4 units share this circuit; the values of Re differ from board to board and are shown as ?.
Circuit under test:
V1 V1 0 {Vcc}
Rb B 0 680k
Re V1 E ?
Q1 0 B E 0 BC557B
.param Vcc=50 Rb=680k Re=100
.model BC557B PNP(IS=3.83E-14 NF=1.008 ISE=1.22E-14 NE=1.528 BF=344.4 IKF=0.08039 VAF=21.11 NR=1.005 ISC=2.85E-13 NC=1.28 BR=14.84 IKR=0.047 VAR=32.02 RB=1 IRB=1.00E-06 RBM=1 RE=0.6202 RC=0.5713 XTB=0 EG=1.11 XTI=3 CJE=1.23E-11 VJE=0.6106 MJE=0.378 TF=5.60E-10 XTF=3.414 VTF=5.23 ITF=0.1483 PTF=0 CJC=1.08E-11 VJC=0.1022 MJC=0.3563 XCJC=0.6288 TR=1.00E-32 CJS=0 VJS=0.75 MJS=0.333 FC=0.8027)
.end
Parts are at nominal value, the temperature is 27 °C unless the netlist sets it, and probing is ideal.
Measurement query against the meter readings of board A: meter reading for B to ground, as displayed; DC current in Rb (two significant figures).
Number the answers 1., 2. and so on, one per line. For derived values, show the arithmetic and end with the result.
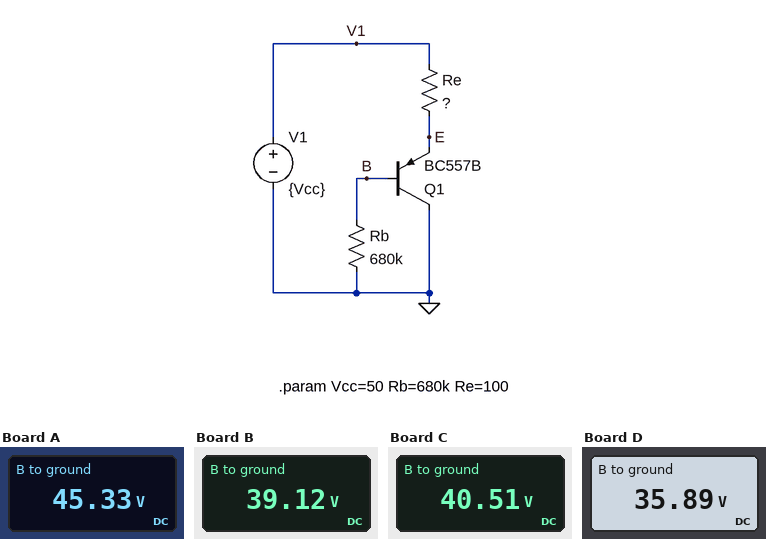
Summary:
1. 45.33 V
2. (45.33 V) / 680 kΩ = 67 µA
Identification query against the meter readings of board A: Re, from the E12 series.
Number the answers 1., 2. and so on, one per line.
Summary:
1. 68 Ω
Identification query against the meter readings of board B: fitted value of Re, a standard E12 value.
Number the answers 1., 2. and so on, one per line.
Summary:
1. 220 Ω
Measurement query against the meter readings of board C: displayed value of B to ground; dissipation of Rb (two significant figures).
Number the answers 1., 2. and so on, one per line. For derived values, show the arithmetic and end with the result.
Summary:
1. 40.51 V
2. (40.51 V)^2 / 680 kΩ = 2.4 mW
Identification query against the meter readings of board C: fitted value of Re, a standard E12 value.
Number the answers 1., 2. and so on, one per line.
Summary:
1. 180 Ω
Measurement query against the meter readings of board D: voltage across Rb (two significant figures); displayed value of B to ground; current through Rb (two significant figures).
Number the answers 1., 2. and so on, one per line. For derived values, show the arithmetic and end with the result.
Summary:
1. 35.89 V = 36 V
2. 35.89 V
3. (35.89 V) / 680 kΩ = 53 µA
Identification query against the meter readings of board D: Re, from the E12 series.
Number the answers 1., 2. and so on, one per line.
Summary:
1. 330 Ω
